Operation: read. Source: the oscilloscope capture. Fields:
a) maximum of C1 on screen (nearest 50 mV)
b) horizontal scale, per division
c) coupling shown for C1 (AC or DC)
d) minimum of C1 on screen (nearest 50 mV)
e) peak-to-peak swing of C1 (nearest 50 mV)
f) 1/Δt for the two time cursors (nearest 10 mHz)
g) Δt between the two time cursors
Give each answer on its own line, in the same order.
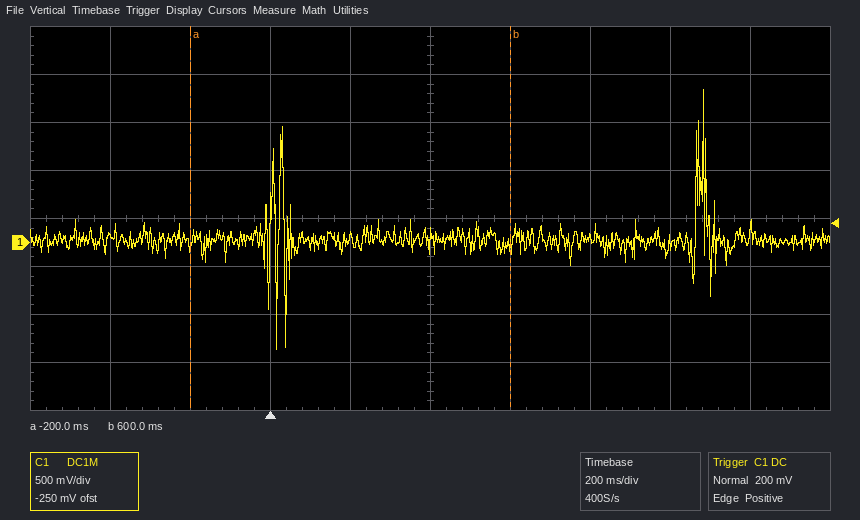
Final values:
1.60 V
200 ms
DC
-1.10 V
2.70 V
1.25 Hz
800 ms
